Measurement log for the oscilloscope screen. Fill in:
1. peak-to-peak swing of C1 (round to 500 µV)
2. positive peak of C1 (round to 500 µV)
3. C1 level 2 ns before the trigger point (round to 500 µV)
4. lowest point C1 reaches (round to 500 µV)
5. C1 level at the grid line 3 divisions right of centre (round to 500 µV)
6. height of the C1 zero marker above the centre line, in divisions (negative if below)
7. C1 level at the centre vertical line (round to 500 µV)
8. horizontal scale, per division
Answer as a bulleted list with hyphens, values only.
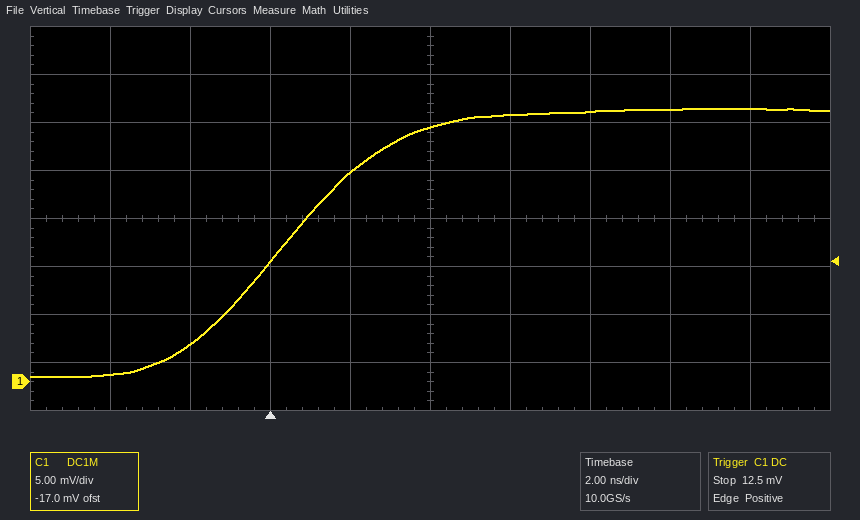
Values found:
- 28.0 mV
- 28.5 mV
- 4.0 mV
- 500 µV
- 28.5 mV
- -3.4 div
- 26.5 mV
- 2 ns
